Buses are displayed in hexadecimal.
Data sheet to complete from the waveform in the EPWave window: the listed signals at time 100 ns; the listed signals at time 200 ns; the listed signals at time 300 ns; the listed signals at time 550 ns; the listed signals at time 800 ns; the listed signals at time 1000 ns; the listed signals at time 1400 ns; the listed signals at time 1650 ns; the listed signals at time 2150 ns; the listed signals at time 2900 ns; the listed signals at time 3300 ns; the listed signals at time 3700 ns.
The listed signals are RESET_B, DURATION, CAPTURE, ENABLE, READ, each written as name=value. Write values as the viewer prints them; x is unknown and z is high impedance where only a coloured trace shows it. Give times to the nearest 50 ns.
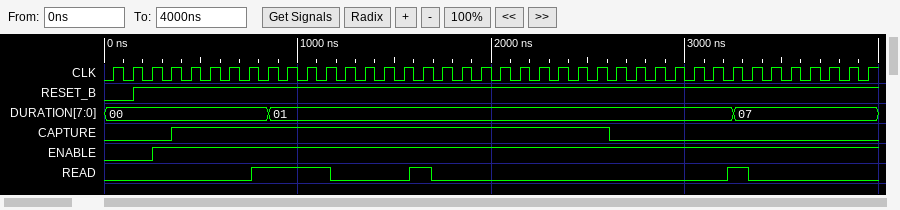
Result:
RESET_B=0, DURATION=00, CAPTURE=0, ENABLE=0, READ=0
RESET_B=1, DURATION=00, CAPTURE=0, ENABLE=0, READ=0
RESET_B=1, DURATION=00, CAPTURE=0, ENABLE=1, READ=0
RESET_B=1, DURATION=00, CAPTURE=1, ENABLE=1, READ=0
RESET_B=1, DURATION=00, CAPTURE=1, ENABLE=1, READ=1
RESET_B=1, DURATION=01, CAPTURE=1, ENABLE=1, READ=1
RESET_B=1, DURATION=01, CAPTURE=1, ENABLE=1, READ=0
RESET_B=1, DURATION=01, CAPTURE=1, ENABLE=1, READ=1
RESET_B=1, DURATION=01, CAPTURE=1, ENABLE=1, READ=0
RESET_B=1, DURATION=01, CAPTURE=0, ENABLE=1, READ=0
RESET_B=1, DURATION=07, CAPTURE=0, ENABLE=1, READ=1
RESET_B=1, DURATION=07, CAPTURE=0, ENABLE=1, READ=0
